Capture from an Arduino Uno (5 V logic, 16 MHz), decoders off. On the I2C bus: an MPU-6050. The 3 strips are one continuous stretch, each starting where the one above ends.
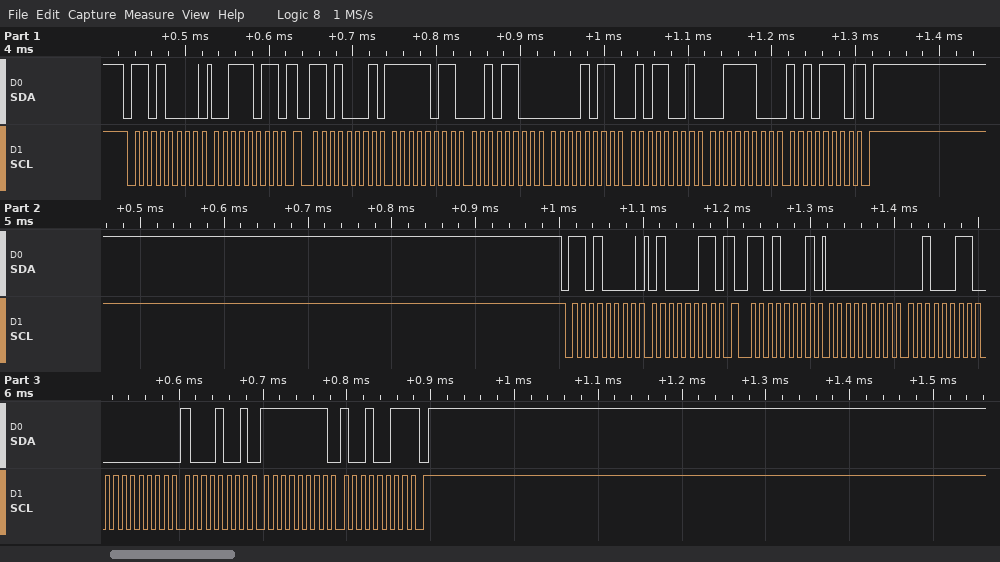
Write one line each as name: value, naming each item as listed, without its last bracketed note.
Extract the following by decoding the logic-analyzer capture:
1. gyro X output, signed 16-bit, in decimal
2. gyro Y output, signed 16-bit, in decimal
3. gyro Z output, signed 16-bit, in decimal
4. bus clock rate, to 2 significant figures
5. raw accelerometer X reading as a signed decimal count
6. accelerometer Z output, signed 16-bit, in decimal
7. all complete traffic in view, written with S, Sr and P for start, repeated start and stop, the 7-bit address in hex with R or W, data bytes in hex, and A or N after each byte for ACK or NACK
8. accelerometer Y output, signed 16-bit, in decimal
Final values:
gyro X output, signed 16-bit, in decimal: 35
gyro Y output, signed 16-bit, in decimal: 137
gyro Z output, signed 16-bit, in decimal: -109
bus clock rate, to 2 significant figures: 100 kHz
raw accelerometer X reading as a signed decimal count: -1236
accelerometer Z output, signed 16-bit, in decimal: 15534
all complete traffic in view, written with S, Sr and P for start, repeated start and stop, the 7-bit address in hex with R or W, data bytes in hex, and A or N after each byte for ACK or NACK: S 68W A 3B A Sr 68R A FB A 2C A 0B A 59 A 3C A AE N P S 68W A 43 A Sr 68R A 00 A 23 A 00 A 89 A FF A 93 N P
accelerometer Y output, signed 16-bit, in decimal: 2905
